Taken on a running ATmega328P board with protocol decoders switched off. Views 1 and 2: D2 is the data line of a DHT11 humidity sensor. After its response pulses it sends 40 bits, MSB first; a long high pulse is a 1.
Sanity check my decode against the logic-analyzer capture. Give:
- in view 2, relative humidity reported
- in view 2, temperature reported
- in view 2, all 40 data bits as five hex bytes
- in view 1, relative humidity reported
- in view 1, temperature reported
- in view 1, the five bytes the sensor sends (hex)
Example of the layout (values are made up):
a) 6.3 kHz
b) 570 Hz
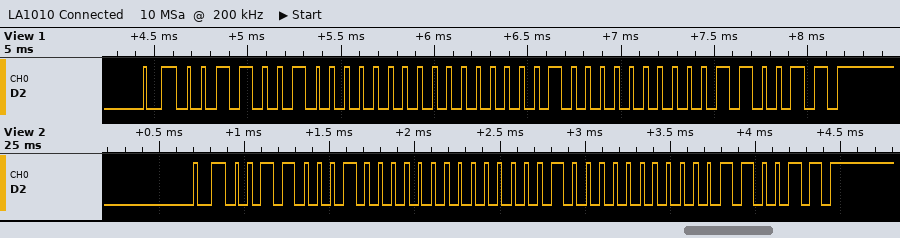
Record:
a) 49 %
b) 2.0 °C
c) 31 00 02 00 33
d) 50 %
e) 1.0 °C
f) 32 00 01 00 33
